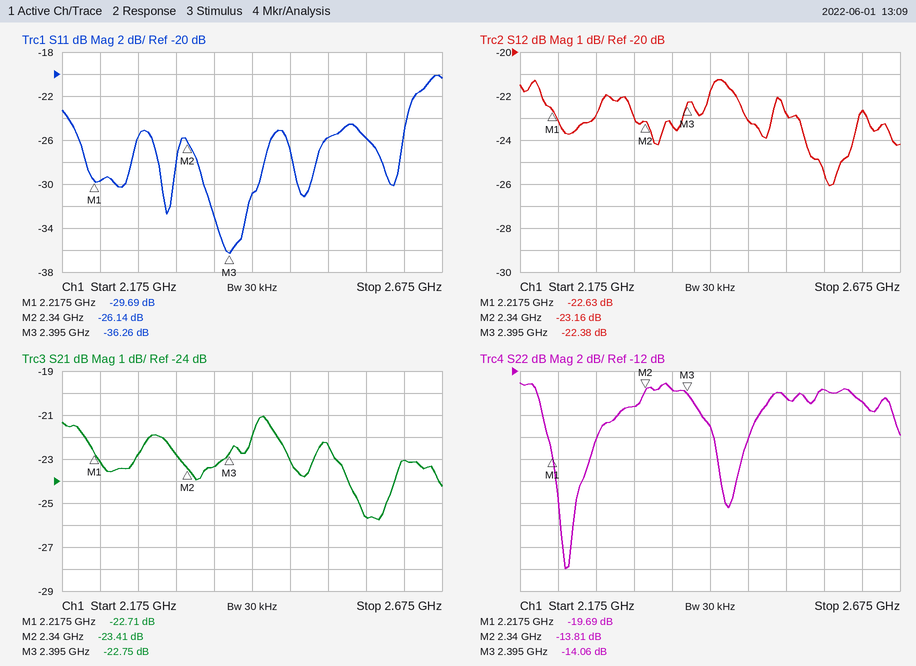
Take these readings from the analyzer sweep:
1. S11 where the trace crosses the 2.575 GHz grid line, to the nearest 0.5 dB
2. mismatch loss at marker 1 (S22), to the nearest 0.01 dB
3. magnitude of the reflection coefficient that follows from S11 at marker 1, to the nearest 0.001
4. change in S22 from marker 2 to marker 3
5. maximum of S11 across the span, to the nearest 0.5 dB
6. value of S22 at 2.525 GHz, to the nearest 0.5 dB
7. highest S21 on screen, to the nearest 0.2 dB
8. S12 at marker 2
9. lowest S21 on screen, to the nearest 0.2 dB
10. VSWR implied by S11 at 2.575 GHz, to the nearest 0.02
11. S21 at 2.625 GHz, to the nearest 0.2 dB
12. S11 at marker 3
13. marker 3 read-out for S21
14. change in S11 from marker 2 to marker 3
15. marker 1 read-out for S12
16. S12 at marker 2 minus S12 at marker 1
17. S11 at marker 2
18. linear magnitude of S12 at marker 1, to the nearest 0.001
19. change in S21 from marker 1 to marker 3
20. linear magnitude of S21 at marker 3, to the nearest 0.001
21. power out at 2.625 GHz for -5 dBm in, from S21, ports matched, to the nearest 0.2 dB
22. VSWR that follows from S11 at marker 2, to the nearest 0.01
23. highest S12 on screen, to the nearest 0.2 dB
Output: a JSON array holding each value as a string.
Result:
["-26.0 dB", "0.05 dB", "0.033", "-0.25 dB", "-20.0 dB", "-14.5 dB", "-21.0 dB", "-23.16 dB", "-25.8 dB", "1.10", "-23.0 dB", "-36.26 dB", "-22.75 dB", "-10.12 dB", "-22.63 dB", "-0.53 dB", "-26.14 dB", "0.074", "-0.04 dB", "0.073", "-28.0 dBm", "1.10", "-21.2 dB"]
